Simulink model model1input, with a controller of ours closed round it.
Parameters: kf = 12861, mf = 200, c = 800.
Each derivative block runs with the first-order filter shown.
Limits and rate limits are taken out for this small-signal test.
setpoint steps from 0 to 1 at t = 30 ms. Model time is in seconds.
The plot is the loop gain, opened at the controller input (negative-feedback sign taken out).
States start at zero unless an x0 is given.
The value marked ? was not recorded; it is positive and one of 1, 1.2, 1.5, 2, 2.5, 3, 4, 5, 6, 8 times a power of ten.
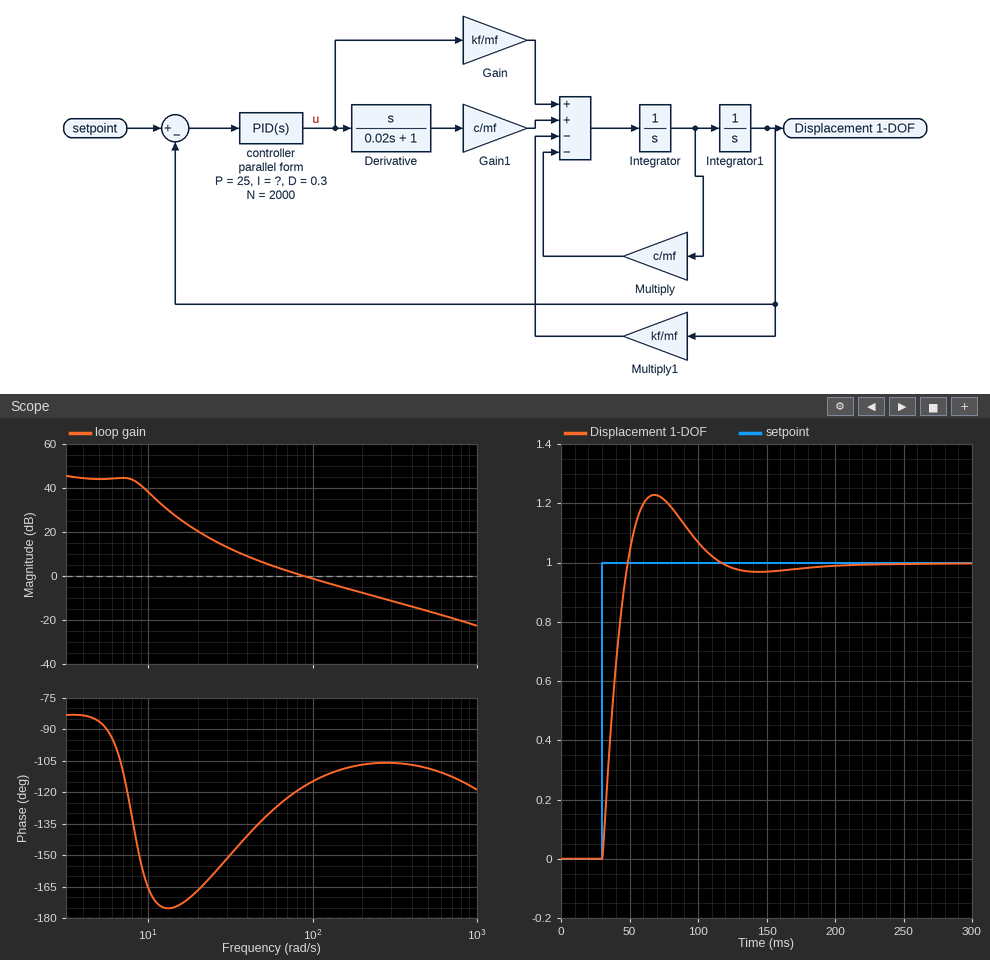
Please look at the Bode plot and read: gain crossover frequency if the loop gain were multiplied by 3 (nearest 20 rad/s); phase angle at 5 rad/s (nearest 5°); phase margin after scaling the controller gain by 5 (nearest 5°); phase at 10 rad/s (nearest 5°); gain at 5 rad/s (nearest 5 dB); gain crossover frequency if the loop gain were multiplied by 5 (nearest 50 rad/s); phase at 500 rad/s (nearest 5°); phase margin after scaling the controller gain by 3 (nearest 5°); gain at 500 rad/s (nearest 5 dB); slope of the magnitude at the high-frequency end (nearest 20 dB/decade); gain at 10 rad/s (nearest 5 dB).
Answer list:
240 rad/s
-85°
75°
-165°
45 dB
400 rad/s
-110°
75°
-15 dB
-20 dB/decade
40 dB
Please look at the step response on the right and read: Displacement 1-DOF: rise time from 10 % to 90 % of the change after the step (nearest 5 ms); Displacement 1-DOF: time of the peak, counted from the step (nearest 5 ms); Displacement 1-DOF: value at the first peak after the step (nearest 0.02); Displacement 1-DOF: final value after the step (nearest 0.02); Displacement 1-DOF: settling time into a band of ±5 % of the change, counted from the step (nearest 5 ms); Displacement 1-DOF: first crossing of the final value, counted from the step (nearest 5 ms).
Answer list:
15 ms
40 ms
1.22
1.00
75 ms
20 ms
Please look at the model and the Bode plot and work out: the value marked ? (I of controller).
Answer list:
500
